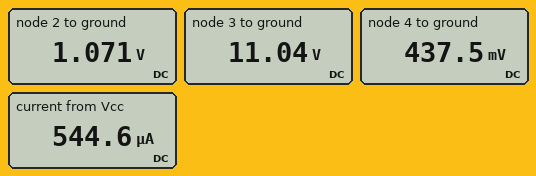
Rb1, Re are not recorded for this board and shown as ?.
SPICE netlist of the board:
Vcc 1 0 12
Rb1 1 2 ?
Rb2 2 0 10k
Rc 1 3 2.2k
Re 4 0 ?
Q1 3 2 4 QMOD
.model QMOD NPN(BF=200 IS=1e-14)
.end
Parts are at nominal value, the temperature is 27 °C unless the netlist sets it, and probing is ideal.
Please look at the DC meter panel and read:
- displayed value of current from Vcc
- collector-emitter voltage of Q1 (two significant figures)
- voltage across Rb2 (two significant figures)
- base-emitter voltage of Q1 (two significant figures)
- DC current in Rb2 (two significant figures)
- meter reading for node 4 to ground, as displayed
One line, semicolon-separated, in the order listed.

544.6 µA; 11 V; 1.1 V; 630 mV; 110 µA; 437.5 mV
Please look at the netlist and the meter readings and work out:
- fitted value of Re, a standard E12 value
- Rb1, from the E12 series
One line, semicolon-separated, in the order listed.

1 kΩ; 100 kΩ
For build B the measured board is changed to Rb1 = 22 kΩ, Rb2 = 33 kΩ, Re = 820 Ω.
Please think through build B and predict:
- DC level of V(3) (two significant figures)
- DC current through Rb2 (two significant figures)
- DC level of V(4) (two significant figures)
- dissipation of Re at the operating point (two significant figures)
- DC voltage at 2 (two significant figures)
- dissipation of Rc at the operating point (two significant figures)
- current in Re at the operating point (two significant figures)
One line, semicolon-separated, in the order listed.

3.5 V; 120 µA; 3.4 V; 14 mW; 4.1 V; 33 mW; 4.1 mA
